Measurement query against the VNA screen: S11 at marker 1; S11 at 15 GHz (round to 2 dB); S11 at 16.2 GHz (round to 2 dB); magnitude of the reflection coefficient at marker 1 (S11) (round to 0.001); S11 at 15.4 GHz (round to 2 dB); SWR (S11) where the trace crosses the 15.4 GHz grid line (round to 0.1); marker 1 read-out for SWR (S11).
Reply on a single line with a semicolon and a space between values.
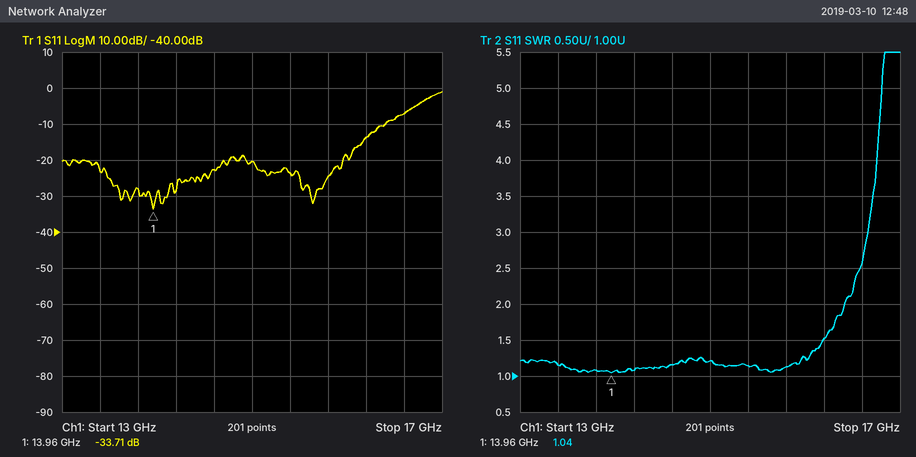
-33.71 dB; -20 dB; -14 dB; 0.021; -24 dB; 1.1; 1.04
